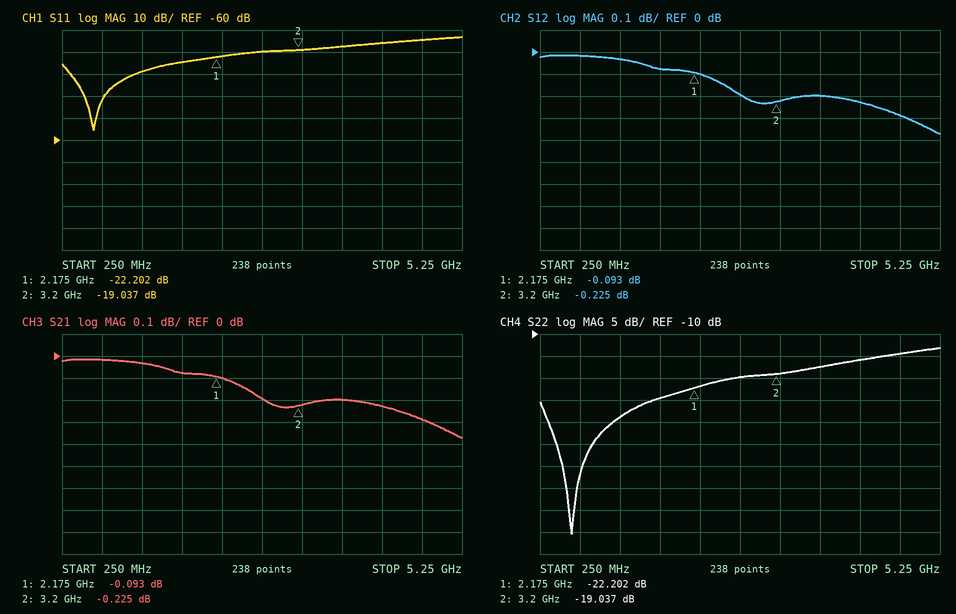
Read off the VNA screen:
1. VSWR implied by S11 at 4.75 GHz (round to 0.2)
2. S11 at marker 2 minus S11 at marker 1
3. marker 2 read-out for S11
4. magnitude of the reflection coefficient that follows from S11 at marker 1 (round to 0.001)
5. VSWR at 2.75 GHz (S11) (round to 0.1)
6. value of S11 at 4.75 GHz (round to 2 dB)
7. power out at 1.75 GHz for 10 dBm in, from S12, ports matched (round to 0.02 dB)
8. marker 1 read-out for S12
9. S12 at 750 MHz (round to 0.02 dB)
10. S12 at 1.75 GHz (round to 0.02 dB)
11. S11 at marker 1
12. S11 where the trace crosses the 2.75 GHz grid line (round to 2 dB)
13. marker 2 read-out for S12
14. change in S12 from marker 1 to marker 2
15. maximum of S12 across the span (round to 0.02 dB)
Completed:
1.4
3.165 dB
-19.037 dB
0.078
1.2
-14 dB
9.92 dBm
-0.093 dB
-0.02 dB
-0.08 dB
-22.202 dB
-20 dB
-0.225 dB
-0.132 dB
-0.02 dB
